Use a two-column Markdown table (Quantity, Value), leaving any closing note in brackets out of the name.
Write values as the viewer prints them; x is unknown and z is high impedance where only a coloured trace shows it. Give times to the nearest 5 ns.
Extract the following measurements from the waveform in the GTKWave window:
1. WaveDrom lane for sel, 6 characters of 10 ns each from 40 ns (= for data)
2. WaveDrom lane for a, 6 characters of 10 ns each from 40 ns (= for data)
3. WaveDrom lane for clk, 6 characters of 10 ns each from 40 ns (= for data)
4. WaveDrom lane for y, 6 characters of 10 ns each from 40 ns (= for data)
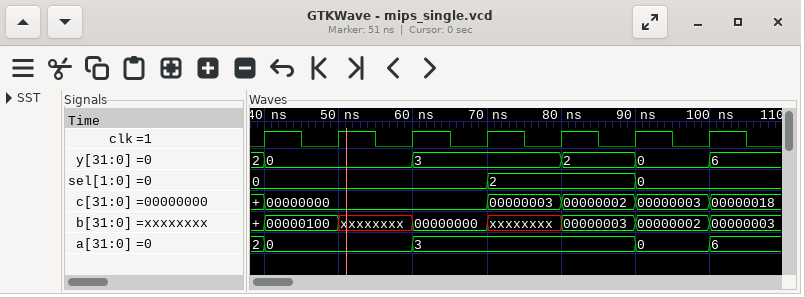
| Quantity | Value |
|---|---|
| WaveDrom lane for sel, 6 characters of 10 ns each from 40 ns | {name: 'sel', wave: '=..=.=', data: '0 2 0'} |
| WaveDrom lane for a, 6 characters of 10 ns each from 40 ns | {name: 'a', wave: '=.=..=', data: '0 3 0'} |
| WaveDrom lane for clk, 6 characters of 10 ns each from 40 ns | {name: 'clk', wave: 'p.....'} |
| WaveDrom lane for y, 6 characters of 10 ns each from 40 ns | {name: 'y', wave: '=.=.==', data: '0 3 2 0'} |
